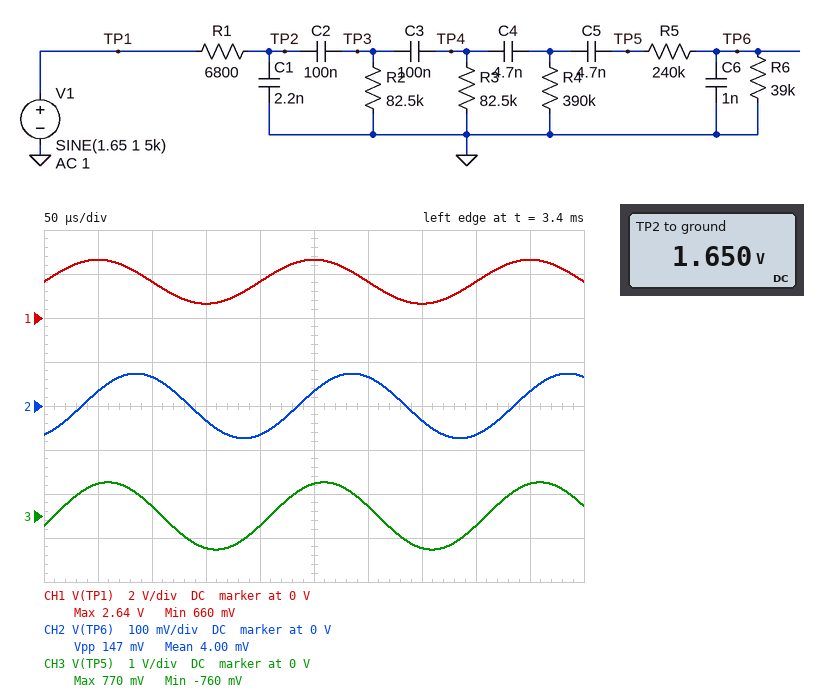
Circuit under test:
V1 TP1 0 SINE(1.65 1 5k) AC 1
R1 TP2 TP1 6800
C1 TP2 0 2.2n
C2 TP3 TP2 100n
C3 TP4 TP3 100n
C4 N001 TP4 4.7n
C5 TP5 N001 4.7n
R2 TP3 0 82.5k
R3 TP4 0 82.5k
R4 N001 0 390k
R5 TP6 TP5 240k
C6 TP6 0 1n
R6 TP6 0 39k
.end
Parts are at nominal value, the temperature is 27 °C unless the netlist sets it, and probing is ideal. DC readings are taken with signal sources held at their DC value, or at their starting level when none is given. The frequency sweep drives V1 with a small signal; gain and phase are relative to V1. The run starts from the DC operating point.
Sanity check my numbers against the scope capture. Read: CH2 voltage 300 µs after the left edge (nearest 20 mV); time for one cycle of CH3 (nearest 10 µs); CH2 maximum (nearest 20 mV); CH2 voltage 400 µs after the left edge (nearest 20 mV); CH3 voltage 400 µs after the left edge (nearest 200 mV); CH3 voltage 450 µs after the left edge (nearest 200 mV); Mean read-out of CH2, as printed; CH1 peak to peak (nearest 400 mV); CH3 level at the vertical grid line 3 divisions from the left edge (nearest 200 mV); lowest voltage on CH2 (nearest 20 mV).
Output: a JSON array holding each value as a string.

["60 mV", "200 µs", "80 mV", "-60 mV", "-200 mV", "800 mV", "4.00 mV", "2.0 V", "-800 mV", "-80 mV"]
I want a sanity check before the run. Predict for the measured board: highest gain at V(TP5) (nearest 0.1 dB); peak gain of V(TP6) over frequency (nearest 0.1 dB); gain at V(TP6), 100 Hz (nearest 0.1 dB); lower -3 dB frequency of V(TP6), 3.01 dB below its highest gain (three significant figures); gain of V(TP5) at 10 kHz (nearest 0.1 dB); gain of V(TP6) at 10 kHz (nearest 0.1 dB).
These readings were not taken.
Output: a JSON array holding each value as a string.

["-1.9 dB", "-19.4 dB", "-30.0 dB", "274 Hz", "-3.7 dB", "-28.2 dB"]
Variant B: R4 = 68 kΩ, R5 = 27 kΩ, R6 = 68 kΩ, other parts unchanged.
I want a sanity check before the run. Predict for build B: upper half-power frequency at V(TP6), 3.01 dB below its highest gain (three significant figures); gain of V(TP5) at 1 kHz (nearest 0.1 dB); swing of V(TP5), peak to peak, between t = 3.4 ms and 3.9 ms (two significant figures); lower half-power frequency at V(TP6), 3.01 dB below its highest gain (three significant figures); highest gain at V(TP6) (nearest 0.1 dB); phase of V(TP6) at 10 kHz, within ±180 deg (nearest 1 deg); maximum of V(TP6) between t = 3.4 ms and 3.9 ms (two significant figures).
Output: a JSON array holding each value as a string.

["7.90 kHz", "-6.6 dB", "1.1 V", "702 Hz", "-8.1 dB", "-75 deg", "350 mV"]
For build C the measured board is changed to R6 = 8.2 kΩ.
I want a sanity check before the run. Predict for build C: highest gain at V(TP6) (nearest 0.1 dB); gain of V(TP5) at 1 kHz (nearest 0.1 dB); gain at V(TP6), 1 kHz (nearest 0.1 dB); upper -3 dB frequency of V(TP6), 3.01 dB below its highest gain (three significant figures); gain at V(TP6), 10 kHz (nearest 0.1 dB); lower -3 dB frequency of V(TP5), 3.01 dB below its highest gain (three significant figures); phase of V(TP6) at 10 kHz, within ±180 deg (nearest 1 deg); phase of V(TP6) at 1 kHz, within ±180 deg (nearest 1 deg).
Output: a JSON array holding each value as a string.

["-31.6 dB", "-2.2 dB", "-31.8 dB", "10.5 kHz", "-34.3 dB", "322 Hz", "-62 deg", "16 deg"]
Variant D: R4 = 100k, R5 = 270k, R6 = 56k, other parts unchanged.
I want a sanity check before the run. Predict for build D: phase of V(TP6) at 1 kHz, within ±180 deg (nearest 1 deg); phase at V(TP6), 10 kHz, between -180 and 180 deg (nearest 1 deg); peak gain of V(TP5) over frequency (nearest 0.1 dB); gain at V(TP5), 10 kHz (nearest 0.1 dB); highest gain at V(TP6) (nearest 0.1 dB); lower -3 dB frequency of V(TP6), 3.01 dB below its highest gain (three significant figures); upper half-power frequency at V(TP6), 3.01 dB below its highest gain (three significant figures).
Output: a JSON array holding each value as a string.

["12 deg", "-104 deg", "-2.4 dB", "-4.0 dB", "-18.6 dB", "386 Hz", "4.04 kHz"]
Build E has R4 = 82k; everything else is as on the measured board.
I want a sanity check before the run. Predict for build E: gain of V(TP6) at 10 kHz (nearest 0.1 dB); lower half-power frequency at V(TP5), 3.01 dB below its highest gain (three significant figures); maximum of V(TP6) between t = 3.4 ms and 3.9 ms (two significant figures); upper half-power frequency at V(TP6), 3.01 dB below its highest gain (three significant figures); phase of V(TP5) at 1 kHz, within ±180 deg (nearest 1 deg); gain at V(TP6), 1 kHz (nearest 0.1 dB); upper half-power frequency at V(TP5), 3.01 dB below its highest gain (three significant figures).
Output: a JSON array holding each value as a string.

["-28.5 dB", "530 Hz", "70 mV", "5.19 kHz", "33 deg", "-20.7 dB", "14.8 kHz"]
